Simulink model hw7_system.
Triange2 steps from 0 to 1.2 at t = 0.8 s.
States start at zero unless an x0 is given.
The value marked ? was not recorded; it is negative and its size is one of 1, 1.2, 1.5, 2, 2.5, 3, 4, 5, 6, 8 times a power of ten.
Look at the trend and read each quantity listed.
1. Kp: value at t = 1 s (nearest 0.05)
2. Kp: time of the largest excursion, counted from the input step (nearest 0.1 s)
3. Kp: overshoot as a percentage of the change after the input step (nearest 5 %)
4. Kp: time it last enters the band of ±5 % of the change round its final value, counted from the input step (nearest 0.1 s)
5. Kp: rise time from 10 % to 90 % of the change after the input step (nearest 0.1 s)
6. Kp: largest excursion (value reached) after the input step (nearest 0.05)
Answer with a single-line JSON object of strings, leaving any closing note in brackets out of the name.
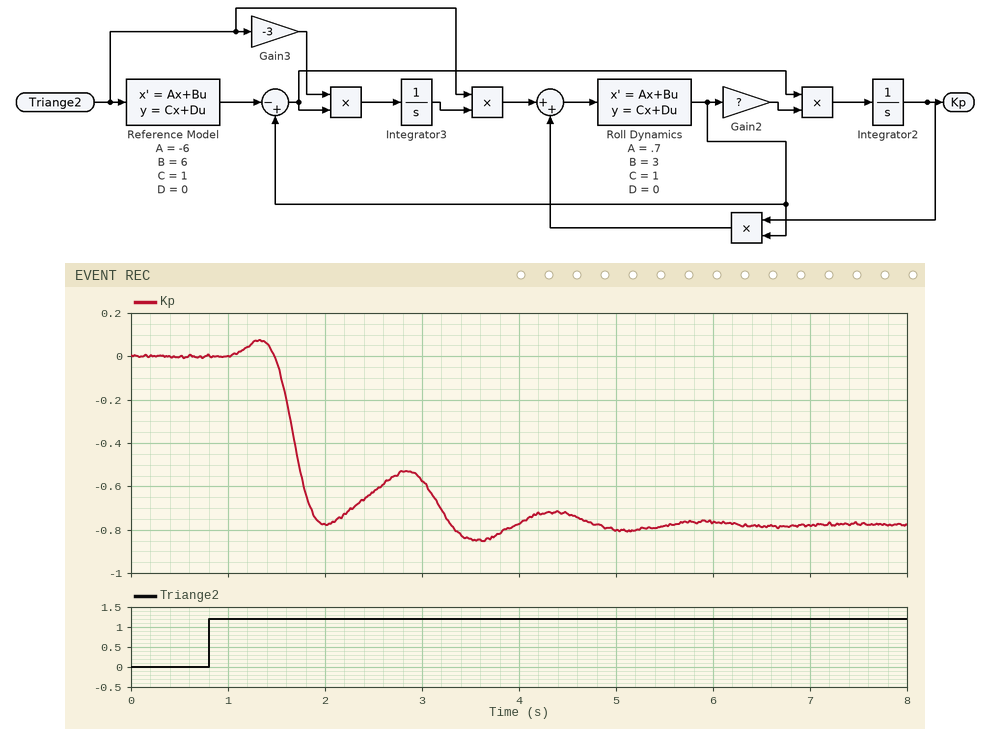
{"Kp: value at t = 1 s": "0.00", "Kp: time of the largest excursion, counted from the input step": "2.8 s", "Kp: overshoot as a percentage of the change after the input step": "10 %", "Kp: time it last enters the band of ±5 % of the change round its final value, counted from the input step": "3.8 s", "Kp: rise time from 10 % to 90 % of the change after the input step": "0.3 s", "Kp: largest excursion (value reached) after the input step": "-0.85"}
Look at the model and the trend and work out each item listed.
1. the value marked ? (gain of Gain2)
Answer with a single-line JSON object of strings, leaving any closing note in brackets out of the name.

{"the value marked ?": "-1"}
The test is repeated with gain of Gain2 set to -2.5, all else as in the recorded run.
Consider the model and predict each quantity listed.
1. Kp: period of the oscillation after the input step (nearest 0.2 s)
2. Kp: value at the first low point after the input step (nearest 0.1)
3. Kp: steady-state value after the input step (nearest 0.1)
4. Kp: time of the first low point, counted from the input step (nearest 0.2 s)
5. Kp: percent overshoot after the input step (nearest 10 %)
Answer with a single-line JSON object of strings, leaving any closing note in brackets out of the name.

{"Kp: period of the oscillation after the input step": "1.4 s", "Kp: value at the first low point after the input step": "-1.2", "Kp: steady-state value after the input step": "-0.9", "Kp: time of the first low point, counted from the input step": "1.0 s", "Kp: percent overshoot after the input step": "30 %"}
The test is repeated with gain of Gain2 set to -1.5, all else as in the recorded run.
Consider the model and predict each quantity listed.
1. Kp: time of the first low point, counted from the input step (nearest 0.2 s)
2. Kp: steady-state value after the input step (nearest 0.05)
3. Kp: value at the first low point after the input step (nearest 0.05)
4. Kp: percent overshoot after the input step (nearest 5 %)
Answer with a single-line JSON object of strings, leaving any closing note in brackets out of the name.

{"Kp: time of the first low point, counted from the input step": "1.2 s", "Kp: steady-state value after the input step": "-0.85", "Kp: value at the first low point after the input step": "-0.95", "Kp: percent overshoot after the input step": "10 %"}
